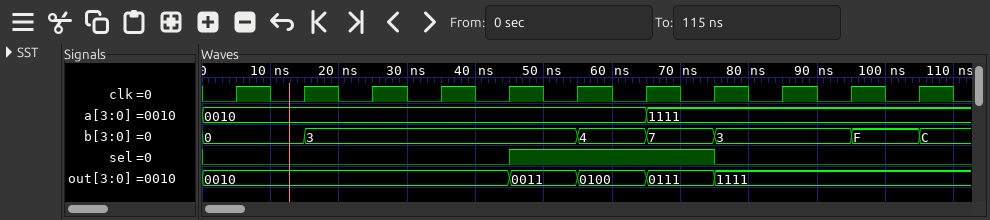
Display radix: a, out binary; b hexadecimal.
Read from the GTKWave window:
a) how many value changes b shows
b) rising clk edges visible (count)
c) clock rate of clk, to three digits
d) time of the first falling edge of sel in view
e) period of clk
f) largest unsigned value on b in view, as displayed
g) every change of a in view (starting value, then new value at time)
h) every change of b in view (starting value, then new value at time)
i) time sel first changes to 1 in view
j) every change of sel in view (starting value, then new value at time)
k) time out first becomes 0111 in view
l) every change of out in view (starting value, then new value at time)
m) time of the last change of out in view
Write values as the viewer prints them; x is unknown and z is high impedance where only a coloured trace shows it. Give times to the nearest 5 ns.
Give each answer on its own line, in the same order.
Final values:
6
11
100 MHz
75 ns
10 ns
F
0010, 1111 at 65 ns
0, 3 at 15 ns, 4 at 55 ns, 7 at 65 ns, 3 at 75 ns, F at 95 ns, C at 105 ns
45 ns
0, 1 at 45 ns, 0 at 75 ns
65 ns
0010, 0011 at 45 ns, 0100 at 55 ns, 0111 at 65 ns, 1111 at 75 ns
75 ns
